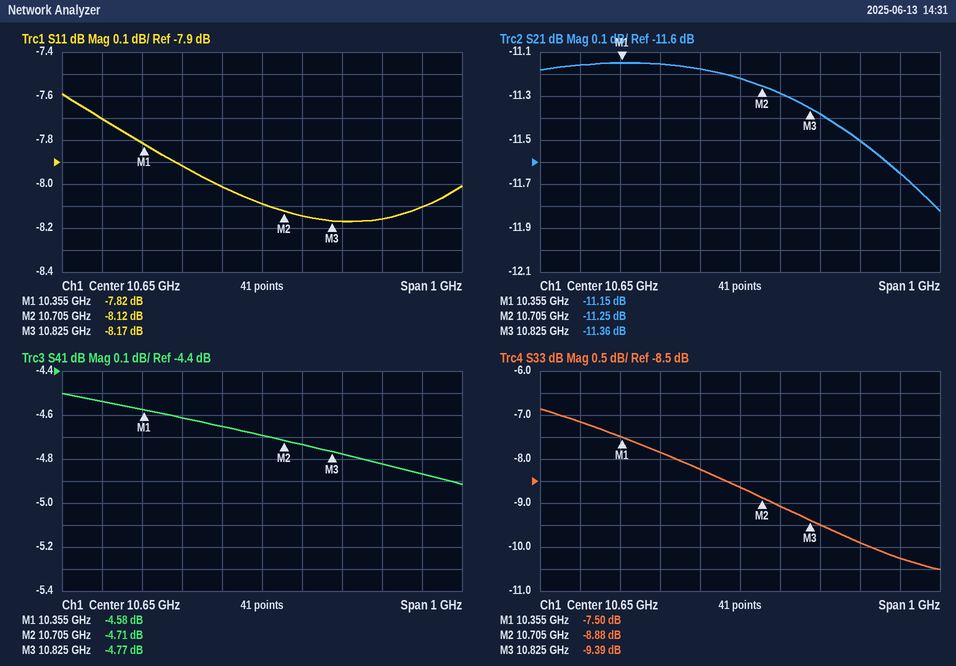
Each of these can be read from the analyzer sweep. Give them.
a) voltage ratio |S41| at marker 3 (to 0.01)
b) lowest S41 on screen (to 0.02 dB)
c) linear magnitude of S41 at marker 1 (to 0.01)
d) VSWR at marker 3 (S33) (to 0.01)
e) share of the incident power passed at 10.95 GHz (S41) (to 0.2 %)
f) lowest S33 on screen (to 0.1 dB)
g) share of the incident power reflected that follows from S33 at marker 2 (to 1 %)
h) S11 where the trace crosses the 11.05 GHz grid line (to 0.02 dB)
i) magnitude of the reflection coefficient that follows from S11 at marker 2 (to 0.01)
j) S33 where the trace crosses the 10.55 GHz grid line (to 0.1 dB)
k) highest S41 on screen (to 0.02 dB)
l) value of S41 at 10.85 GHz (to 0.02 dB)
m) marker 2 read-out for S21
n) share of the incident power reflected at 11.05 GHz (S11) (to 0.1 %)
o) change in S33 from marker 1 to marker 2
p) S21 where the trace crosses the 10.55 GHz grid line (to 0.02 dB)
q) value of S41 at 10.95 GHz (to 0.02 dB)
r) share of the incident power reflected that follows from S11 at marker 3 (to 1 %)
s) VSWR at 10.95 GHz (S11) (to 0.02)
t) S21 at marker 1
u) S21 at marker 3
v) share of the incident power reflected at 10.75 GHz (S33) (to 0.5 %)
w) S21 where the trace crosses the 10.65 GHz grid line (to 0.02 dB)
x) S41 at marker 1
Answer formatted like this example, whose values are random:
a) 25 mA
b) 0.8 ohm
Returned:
a) 0.58
b) -4.92 dB
c) 0.59
d) 2.03
e) 33.0 %
f) -10.5 dB
g) 13 %
h) -8.10 dB
i) 0.39
j) -8.2 dB
k) -4.50 dB
l) -4.78 dB
m) -11.25 dB
n) 15.5 %
o) -1.38 dB
p) -11.18 dB
q) -4.82 dB
r) 15 %
s) 2.28
t) -11.15 dB
u) -11.36 dB
v) 12.5 %
w) -11.22 dB
x) -4.58 dB
